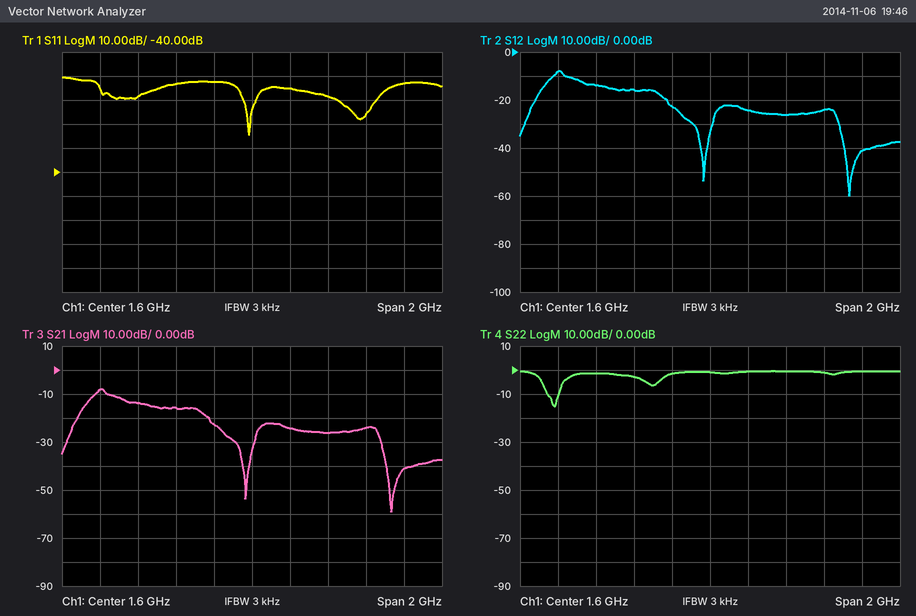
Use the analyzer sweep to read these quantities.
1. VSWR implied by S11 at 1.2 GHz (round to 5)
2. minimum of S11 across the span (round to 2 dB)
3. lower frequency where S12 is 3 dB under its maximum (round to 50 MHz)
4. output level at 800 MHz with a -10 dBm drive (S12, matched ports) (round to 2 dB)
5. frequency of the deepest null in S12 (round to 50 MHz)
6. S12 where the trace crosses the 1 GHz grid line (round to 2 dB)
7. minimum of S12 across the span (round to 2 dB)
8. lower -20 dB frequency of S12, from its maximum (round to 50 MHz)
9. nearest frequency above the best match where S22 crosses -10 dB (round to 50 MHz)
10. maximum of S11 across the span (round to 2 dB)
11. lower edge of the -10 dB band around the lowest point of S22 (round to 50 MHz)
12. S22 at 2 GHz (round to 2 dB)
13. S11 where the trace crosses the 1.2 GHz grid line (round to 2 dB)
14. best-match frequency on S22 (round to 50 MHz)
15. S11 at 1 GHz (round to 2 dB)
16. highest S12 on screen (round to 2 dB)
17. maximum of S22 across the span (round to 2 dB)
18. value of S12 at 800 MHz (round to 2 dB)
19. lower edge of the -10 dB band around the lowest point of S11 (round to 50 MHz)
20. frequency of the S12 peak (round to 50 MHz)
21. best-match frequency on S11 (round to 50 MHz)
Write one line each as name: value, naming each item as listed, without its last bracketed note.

VSWR implied by S11 at 1.2 GHz: 5
minimum of S11 across the span: -24 dB
lower frequency where S12 is 3 dB under its maximum: 750 MHz
output level at 800 MHz with a -10 dBm drive (S12, matched ports): -18 dBm
frequency of the deepest null in S12: 2.35 GHz
S12 where the trace crosses the 1 GHz grid line: -14 dB
minimum of S12 across the span: -60 dB
lower -20 dB frequency of S12, from its maximum: 650 MHz
nearest frequency above the best match where S22 crosses -10 dB: 800 MHz
maximum of S11 across the span: 0 dB
lower edge of the -10 dB band around the lowest point of S22: 750 MHz
S22 at 2 GHz: 0 dB
S11 where the trace crosses the 1.2 GHz grid line: -4 dB
best-match frequency on S22: 800 MHz
S11 at 1 GHz: -8 dB
highest S12 on screen: -8 dB
maximum of S22 across the span: 0 dB
value of S12 at 800 MHz: -8 dB
lower edge of the -10 dB band around the lowest point of S11: 1.55 GHz
frequency of the S12 peak: 800 MHz
best-match frequency on S11: 1.60 GHz
